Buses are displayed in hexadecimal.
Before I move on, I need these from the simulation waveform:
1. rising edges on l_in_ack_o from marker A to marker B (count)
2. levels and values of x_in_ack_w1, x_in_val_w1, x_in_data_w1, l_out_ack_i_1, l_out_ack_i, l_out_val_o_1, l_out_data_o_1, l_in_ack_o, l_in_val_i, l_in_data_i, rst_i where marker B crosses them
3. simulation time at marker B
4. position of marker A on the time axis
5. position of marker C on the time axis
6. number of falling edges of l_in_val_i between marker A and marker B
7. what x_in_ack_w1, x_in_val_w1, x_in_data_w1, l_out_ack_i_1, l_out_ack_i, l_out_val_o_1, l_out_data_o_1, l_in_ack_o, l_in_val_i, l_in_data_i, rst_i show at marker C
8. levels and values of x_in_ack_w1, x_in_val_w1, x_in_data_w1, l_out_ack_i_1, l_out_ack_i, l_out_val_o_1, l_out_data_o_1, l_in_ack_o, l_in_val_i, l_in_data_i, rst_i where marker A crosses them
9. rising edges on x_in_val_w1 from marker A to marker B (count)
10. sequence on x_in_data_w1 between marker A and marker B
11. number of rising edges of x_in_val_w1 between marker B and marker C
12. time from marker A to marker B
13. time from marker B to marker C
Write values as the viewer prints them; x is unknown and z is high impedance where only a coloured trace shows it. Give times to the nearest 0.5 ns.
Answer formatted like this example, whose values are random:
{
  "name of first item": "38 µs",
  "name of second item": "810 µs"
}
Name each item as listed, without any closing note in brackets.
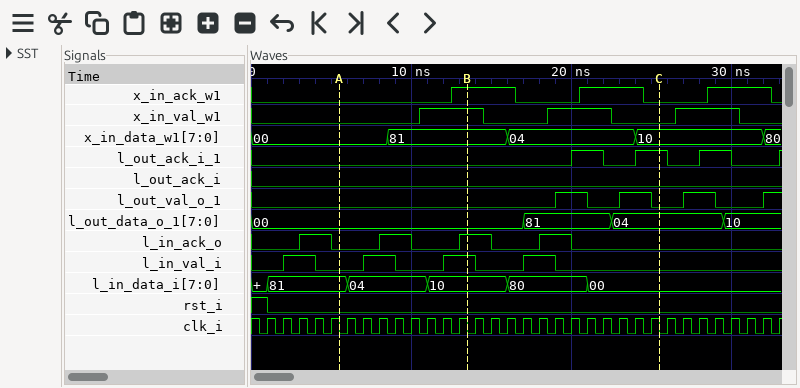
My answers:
{
  "rising edges on l_in_ack_o from marker A to marker B": "2",
  "levels and values of x_in_ack_w1, x_in_val_w1, x_in_data_w1, l_out_ack_i_1, l_out_ack_i, l_out_val_o_1, l_out_data_o_1, l_in_ack_o, l_in_val_i, l_in_data_i, rst_i where marker B crosses them": "x_in_ack_w1=1, x_in_val_w1=1, x_in_data_w1=81, l_out_ack_i_1=0, l_out_ack_i=0, l_out_val_o_1=0, l_out_data_o_1=00, l_in_ack_o=1, l_in_val_i=1, l_in_data_i=10, rst_i=0",
  "simulation time at marker B": "13.5 ns",
  "position of marker A on the time axis": "5.5 ns",
  "position of marker C on the time axis": "25.5 ns",
  "number of falling edges of l_in_val_i between marker A and marker B": "1",
  "what x_in_ack_w1, x_in_val_w1, x_in_data_w1, l_out_ack_i_1, l_out_ack_i, l_out_val_o_1, l_out_data_o_1, l_in_ack_o, l_in_val_i, l_in_data_i, rst_i show at marker C": "x_in_ack_w1=0, x_in_val_w1=0, x_in_data_w1=10, l_out_ack_i_1=1, l_out_ack_i=0, l_out_val_o_1=0, l_out_data_o_1=04, l_in_ack_o=0, l_in_val_i=0, l_in_data_i=00, rst_i=0",
  "levels and values of x_in_ack_w1, x_in_val_w1, x_in_data_w1, l_out_ack_i_1, l_out_ack_i, l_out_val_o_1, l_out_data_o_1, l_in_ack_o, l_in_val_i, l_in_data_i, rst_i where marker A crosses them": "x_in_ack_w1=0, x_in_val_w1=0, x_in_data_w1=00, l_out_ack_i_1=0, l_out_ack_i=0, l_out_val_o_1=0, l_out_data_o_1=00, l_in_ack_o=0, l_in_val_i=0, l_in_data_i=81, rst_i=0",
  "rising edges on x_in_val_w1 from marker A to marker B": "1",
  "sequence on x_in_data_w1 between marker A and marker B": "00, 81",
  "number of rising edges of x_in_val_w1 between marker B and marker C": "1",
  "time from marker A to marker B": "8 ns",
  "time from marker B to marker C": "12 ns"
}
